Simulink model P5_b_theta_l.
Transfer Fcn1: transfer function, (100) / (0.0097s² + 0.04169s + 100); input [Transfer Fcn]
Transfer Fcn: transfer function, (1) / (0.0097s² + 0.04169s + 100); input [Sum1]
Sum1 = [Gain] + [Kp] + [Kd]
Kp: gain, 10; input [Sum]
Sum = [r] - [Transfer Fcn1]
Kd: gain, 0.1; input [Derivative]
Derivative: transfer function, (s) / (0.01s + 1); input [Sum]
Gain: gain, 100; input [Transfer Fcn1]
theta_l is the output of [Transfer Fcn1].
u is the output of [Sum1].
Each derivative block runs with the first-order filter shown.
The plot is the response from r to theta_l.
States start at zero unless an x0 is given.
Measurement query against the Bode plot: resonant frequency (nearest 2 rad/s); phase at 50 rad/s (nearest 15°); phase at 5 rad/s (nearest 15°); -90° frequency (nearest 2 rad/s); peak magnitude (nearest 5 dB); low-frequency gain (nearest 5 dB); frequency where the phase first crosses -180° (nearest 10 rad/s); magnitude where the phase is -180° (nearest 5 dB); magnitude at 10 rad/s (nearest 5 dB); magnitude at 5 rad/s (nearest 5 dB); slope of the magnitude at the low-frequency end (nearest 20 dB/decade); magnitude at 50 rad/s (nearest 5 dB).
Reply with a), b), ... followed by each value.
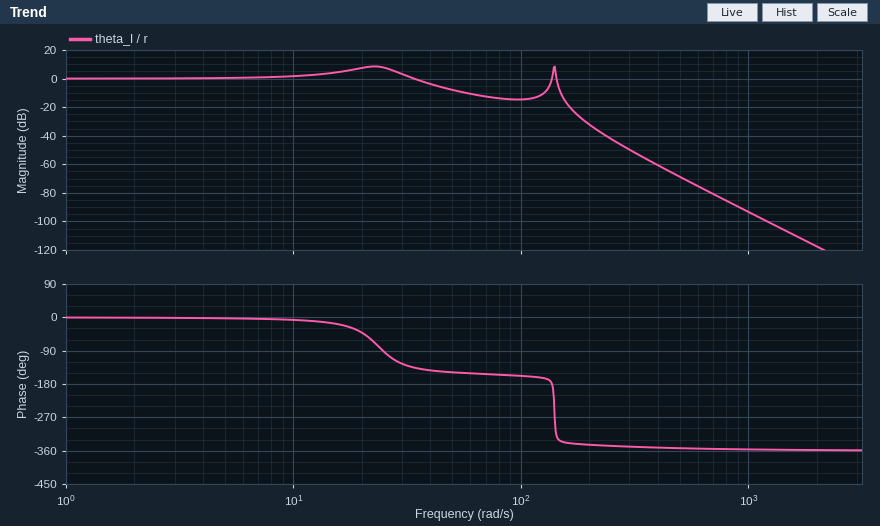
a) 22 rad/s
b) -150°
c) 0°
d) 24 rad/s
e) 10 dB
f) 0 dB
g) 140 rad/s
h) 0 dB
i) 0 dB
j) 0 dB
k) 0 dB/decade
l) -10 dB
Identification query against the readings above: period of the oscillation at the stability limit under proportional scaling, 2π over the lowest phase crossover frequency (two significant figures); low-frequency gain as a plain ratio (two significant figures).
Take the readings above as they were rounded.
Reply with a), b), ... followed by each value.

a) 0.045 s
b) 1.0
